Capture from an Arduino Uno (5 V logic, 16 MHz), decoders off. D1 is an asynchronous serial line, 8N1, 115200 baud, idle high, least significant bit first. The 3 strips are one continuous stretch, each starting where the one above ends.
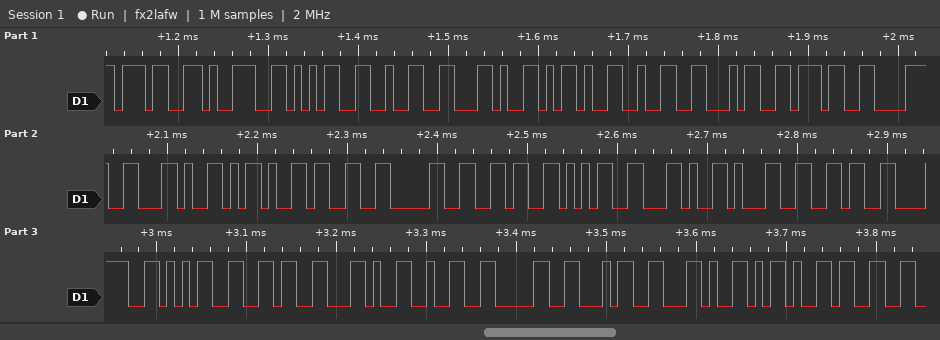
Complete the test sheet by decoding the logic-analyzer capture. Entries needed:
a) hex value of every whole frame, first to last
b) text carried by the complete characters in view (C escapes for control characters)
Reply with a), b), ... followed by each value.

a) 37 39 35 32 2C 2D 32 34 37 38 2C 2D 33 30 36 35 2C 31 36 38 35 36 2C 32 30 34 2C 2D 33
b) "7952,-2478,-3065,16856,204,-3"
